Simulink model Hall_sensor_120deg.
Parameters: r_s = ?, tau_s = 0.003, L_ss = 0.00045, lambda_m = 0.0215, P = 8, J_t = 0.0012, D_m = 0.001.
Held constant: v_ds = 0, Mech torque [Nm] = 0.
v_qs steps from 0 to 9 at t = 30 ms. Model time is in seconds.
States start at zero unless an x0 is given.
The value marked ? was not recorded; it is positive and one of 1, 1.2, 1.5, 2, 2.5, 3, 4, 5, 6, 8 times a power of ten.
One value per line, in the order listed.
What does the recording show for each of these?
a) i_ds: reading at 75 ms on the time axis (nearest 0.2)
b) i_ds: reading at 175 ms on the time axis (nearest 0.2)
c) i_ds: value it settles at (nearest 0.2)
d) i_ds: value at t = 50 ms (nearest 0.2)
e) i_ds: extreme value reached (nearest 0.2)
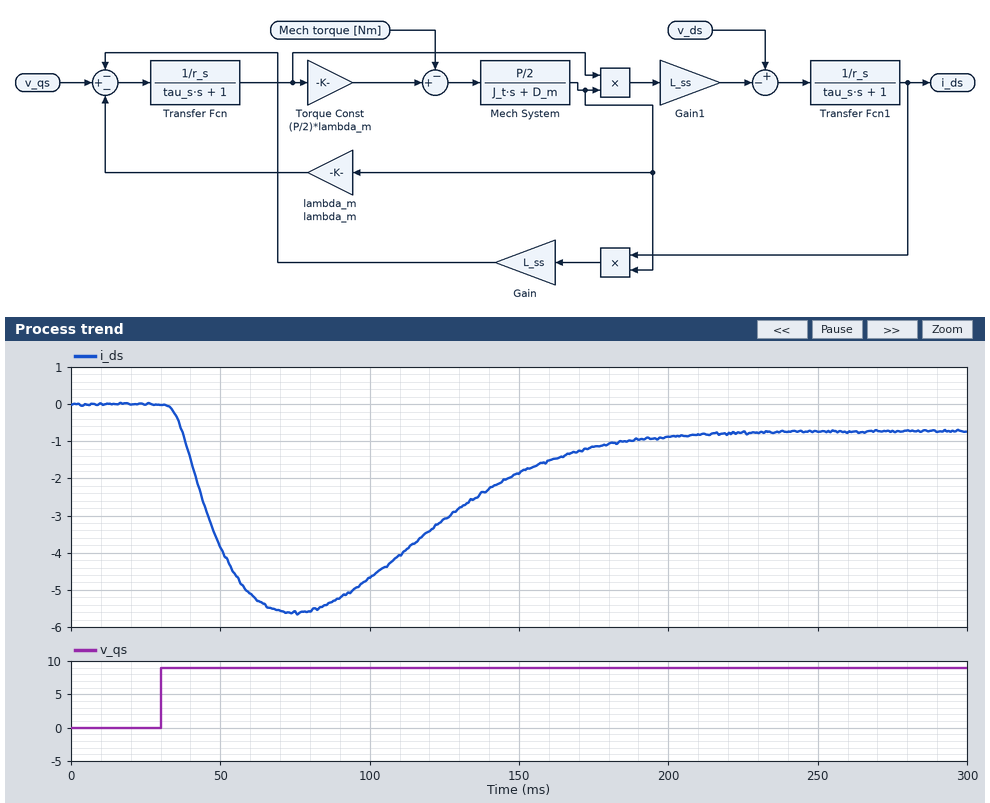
-5.6
-1.2
-0.8
-3.8
-5.6
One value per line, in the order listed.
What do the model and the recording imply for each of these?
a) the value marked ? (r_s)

0.3
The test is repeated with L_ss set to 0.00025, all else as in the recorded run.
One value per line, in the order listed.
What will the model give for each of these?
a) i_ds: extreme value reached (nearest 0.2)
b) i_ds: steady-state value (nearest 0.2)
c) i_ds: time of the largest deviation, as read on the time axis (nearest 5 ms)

-2.8
-0.4
70 ms
